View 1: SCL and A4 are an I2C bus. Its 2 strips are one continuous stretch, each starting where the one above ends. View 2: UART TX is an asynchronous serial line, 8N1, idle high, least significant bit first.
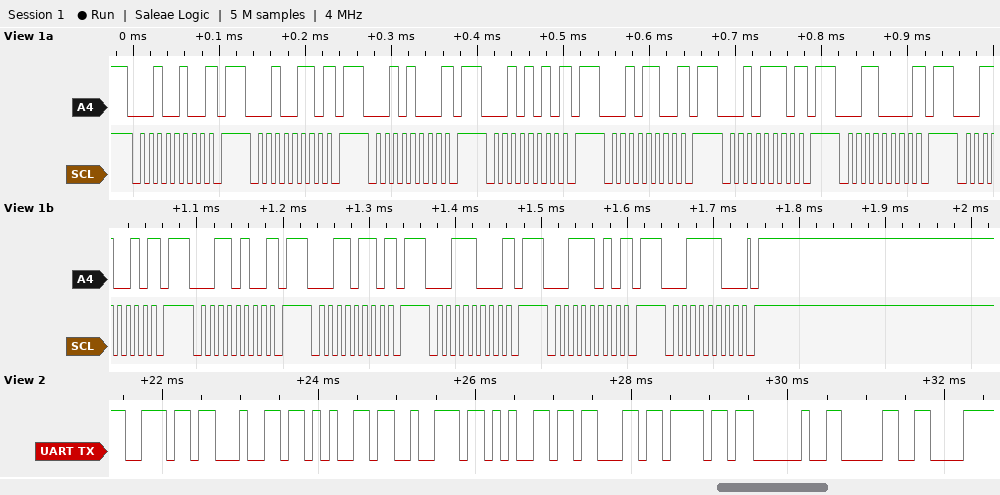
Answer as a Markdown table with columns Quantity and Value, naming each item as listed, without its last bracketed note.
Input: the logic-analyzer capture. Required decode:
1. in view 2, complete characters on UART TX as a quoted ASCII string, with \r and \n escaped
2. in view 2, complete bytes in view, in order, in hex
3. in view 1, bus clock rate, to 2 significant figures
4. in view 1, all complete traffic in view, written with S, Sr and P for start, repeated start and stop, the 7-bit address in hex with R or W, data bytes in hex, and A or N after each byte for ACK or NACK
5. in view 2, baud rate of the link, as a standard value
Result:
| Quantity | Value |
|---|---|
| in view 2, complete characters on UART TX as a quoted ASCII string, with \r and \n escaped | "ndereco 0" |
| in view 2, complete bytes in view, in order, in hex | 6E 64 65 72 65 63 6F 20 30 |
| in view 1, bus clock rate, to 2 significant figures | 100 kHz |
| in view 1, all complete traffic in view, written with S, Sr and P for start, repeated start and stop, the 7-bit address in hex with R or W, data bytes in hex, and A or N after each byte for ACK or NACK | S 12W N P S 13W N P S 14W N P S 15W N P S 16W N P S 17W N P S 18W N P S 19W N P S 1AW N P S 1BW N P S 1CW N P S 1DW N P S 1EW A P |
| in view 2, baud rate of the link, as a standard value | 9600 baud |
